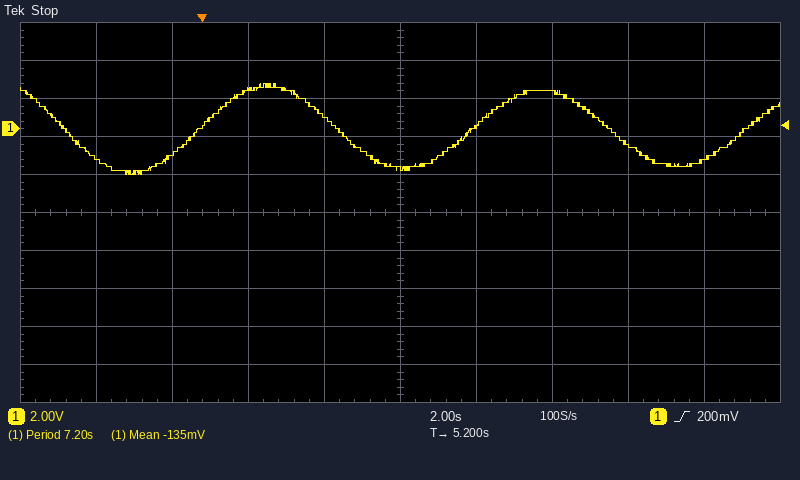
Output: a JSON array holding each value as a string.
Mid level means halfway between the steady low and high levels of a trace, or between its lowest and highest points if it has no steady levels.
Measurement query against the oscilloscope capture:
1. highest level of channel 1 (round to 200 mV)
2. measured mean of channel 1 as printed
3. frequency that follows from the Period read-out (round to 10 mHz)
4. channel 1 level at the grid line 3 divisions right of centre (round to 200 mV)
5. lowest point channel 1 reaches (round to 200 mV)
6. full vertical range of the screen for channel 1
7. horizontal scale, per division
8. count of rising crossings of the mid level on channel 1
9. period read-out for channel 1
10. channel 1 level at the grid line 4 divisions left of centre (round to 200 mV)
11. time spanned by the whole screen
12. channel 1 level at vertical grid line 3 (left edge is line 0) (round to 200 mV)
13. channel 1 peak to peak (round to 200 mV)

["2.4 V", "-135 mV", "140 mHz", "-800 mV", "-2.4 V", "20 V", "2 s", "3", "7.20 s", "-1.6 V", "20 s", "2.0 V", "4.8 V"]
